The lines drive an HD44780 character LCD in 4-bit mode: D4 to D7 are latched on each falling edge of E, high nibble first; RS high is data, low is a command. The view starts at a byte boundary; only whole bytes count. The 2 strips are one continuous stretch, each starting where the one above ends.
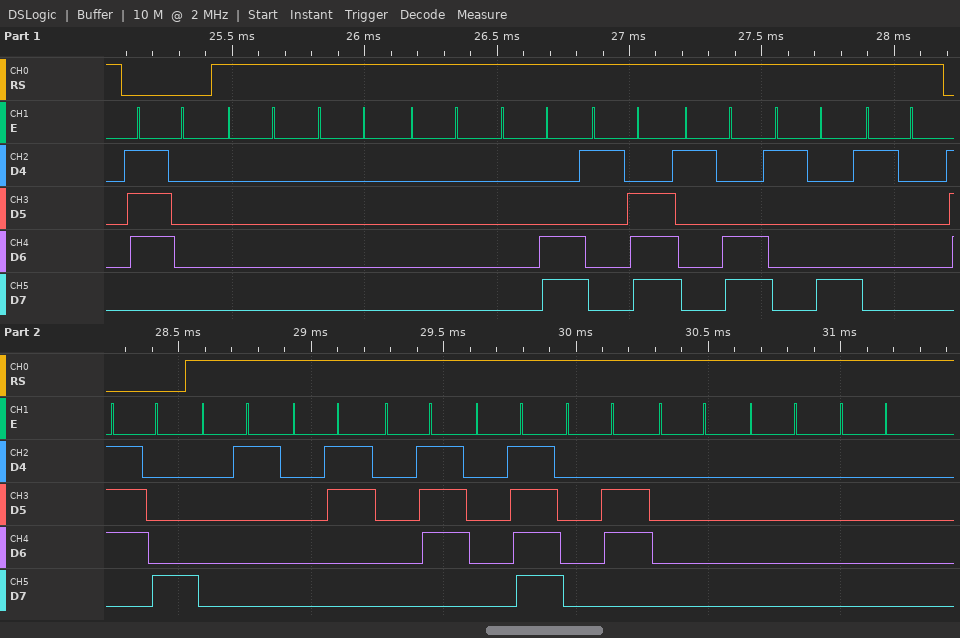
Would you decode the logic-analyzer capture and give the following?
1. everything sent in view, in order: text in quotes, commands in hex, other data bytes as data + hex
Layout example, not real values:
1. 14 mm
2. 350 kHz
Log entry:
1. 0x70 data 00 00 00 0C 1E 1C 18 10 0x78 data 01 03 07 0F 06 00 00 00
